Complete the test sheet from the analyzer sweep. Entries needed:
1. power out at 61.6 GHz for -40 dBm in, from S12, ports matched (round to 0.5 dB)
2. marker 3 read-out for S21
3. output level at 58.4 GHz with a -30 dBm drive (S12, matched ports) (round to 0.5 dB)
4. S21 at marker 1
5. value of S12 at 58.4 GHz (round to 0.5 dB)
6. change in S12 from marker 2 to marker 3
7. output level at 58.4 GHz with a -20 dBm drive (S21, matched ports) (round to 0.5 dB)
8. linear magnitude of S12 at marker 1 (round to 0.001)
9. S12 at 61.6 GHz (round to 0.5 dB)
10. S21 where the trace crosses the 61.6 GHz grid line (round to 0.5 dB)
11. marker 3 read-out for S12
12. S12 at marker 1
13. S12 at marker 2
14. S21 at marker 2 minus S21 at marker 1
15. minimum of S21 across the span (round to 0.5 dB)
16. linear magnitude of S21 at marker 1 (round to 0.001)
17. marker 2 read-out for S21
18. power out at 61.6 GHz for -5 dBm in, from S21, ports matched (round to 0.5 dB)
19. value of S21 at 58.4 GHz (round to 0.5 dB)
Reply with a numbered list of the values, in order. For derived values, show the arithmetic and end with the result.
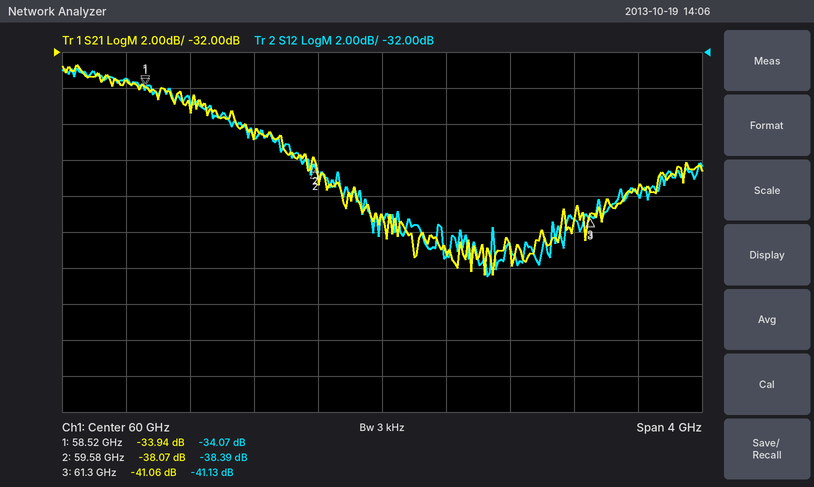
1. -40 dBm + (-40.0 dB) = -80.0 dBm
2. -41.06 dB
3. -30 dBm + (-33.5 dB) = -63.5 dBm
4. -33.94 dB
5. -33.5 dB
6. -41.13 − (-38.39) = -2.74 dB
7. -20 dBm + (-33.5 dB) = -53.5 dBm
8. 10^(-34.07/20) ≈ 0.020
9. -40.0 dB
10. -39.5 dB
11. -41.13 dB
12. -34.07 dB
13. -38.39 dB
14. -38.07 − (-33.94) = -4.13 dB
15. -44.5 dB
16. 10^(-33.94/20) ≈ 0.020
17. -38.07 dB
18. -5 dBm + (-39.5 dB) = -44.5 dBm
19. -33.5 dB
